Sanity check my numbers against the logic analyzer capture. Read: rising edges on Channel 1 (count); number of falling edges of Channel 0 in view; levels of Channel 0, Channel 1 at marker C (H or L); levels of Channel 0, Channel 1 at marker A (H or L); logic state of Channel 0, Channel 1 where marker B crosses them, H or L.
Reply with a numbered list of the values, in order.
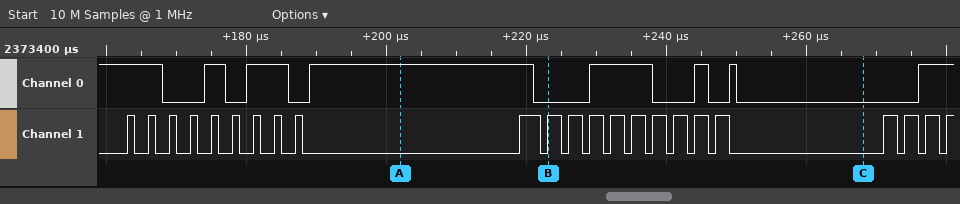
1. 23
2. 7
3. Channel 0=L, Channel 1=L
4. Channel 0=H, Channel 1=L
5. Channel 0=L, Channel 1=H
